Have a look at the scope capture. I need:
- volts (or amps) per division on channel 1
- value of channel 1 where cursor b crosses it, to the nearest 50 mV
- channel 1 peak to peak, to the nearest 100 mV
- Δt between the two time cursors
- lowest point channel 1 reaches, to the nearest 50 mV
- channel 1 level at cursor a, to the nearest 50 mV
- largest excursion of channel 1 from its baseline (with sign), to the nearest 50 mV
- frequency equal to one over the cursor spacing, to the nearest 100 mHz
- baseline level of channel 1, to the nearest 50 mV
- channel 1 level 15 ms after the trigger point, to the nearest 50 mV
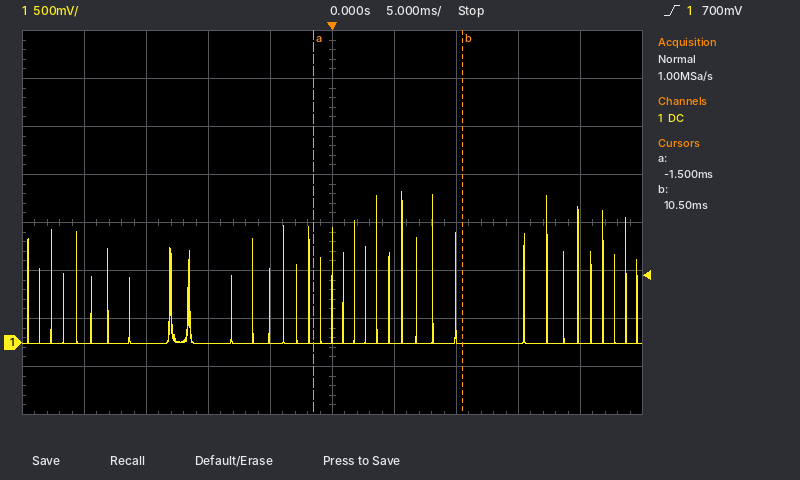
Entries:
500 mV
0 mV
1.60 V
12.0 ms
0 mV
0 mV
+1.60 V
83.3 Hz
0 mV
0 mV
